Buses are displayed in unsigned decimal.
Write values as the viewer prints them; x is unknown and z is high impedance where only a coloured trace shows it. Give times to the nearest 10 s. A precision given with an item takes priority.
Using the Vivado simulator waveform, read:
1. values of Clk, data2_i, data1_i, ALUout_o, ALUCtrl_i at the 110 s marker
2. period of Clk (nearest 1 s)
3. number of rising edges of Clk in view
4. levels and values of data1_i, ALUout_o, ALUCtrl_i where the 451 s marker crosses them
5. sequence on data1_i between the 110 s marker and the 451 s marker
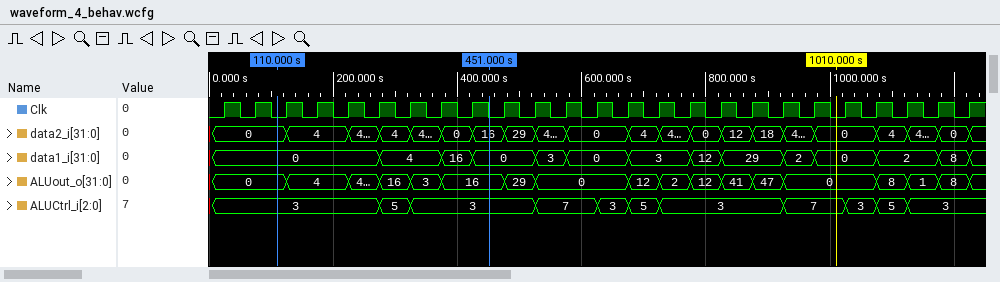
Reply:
Clk=0, data2_i=0, data1_i=0, ALUout_o=0, ALUCtrl_i=3
50 s
25
data1_i=0, ALUout_o=16, ALUCtrl_i=3
0, 4, 16, 0
